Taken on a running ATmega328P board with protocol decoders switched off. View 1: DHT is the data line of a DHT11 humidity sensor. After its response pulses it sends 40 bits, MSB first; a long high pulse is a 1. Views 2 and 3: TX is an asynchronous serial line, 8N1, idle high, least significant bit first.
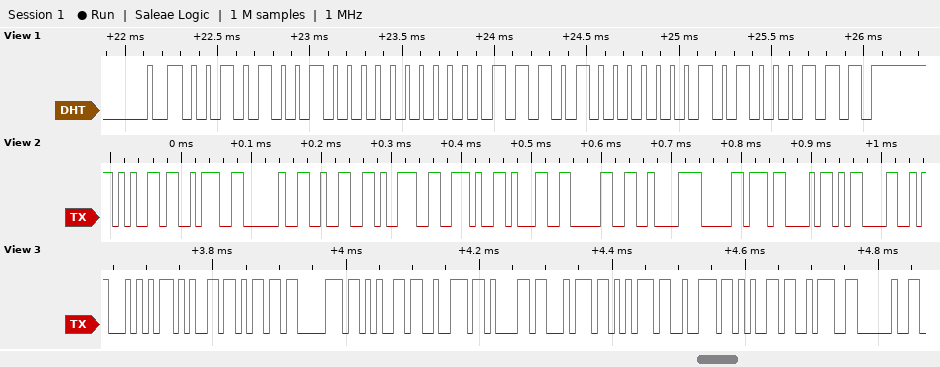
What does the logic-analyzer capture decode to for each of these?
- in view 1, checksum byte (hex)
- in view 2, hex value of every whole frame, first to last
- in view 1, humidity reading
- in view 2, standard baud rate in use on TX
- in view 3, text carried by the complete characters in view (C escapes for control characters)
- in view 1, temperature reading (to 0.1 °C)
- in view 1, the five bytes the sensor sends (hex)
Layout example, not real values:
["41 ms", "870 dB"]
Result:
["0x47", "0x65 0x3A 0x20 0x32 0x39 0x2E 0x31 0x30 0xC2 0xB0 0x43 0x0D", "41 %", "115200 baud", "\"Temperature: \"", "29.1 °C", "29 00 1D 01 47"]
